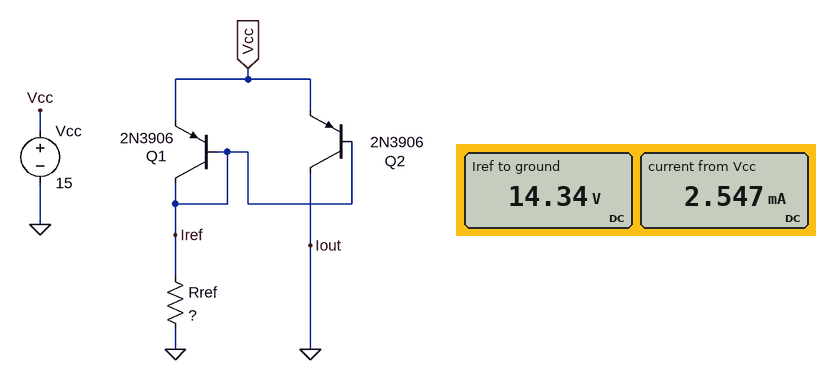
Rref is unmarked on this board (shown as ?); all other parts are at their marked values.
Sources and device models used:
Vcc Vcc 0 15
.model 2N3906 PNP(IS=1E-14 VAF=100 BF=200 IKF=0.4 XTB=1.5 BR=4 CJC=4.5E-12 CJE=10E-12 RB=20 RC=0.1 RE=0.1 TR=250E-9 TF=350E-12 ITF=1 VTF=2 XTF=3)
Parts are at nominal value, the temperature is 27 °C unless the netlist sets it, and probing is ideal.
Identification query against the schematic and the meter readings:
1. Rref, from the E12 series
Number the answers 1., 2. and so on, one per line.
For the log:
1. 12 kΩ
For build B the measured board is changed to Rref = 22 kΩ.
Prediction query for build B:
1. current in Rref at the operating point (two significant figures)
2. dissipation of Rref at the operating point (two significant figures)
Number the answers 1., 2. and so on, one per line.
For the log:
1. 650 µA
2. 9.4 mW
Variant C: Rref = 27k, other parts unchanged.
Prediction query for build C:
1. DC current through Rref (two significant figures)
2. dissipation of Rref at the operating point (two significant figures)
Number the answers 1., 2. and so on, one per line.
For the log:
1. 530 µA
2. 7.6 mW
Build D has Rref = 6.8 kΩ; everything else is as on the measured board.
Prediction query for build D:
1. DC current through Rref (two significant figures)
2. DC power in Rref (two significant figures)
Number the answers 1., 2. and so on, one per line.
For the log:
1. 2.1 mA
2. 30 mW
